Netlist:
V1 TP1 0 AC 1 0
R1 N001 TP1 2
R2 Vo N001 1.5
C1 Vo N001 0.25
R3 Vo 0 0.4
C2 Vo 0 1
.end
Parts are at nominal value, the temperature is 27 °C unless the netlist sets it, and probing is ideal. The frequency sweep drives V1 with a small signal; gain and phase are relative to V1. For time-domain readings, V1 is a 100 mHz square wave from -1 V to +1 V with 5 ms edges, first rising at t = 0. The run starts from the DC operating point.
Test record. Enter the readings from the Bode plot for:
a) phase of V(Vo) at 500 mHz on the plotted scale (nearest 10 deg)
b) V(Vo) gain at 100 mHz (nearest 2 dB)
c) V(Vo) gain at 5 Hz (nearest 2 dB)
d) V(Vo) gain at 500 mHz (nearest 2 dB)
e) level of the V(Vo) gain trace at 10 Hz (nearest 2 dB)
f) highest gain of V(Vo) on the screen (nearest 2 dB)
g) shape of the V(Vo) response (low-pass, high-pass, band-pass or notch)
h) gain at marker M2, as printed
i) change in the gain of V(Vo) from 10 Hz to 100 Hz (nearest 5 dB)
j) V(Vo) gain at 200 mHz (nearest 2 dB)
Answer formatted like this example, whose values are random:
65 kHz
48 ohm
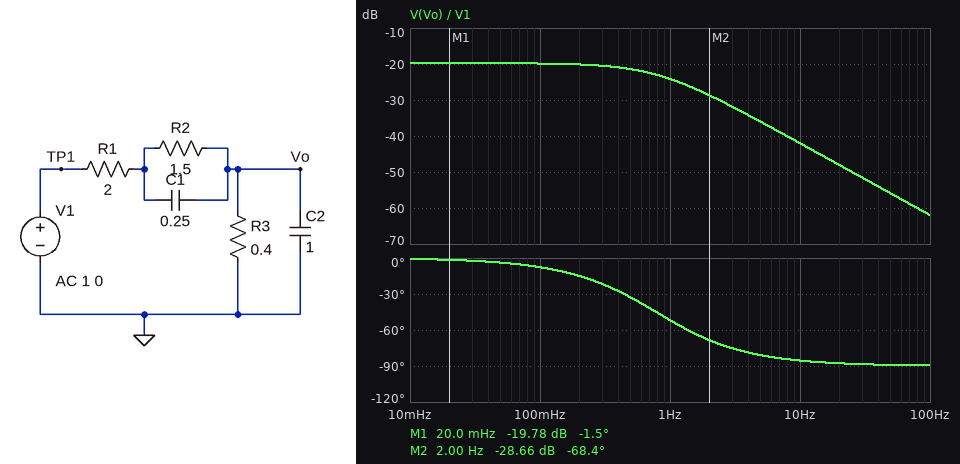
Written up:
-30 deg
-20 dB
-36 dB
-22 dB
-42 dB
-20 dB
low-pass
-28.66 dB
-20 dB
-20 dB
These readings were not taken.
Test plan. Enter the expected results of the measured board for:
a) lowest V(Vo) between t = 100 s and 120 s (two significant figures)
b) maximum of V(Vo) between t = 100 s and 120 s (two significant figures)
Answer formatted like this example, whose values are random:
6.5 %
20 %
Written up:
-100 mV
100 mV
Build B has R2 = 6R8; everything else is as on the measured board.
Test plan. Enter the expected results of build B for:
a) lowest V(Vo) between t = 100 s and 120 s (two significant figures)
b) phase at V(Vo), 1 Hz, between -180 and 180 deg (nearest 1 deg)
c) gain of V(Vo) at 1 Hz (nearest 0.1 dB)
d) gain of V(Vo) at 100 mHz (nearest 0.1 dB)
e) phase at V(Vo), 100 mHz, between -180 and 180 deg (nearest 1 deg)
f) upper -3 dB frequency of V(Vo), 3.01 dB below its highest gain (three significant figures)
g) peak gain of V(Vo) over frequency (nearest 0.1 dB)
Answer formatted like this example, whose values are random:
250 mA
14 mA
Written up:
-120 mV
-48 deg
-23.6 dB
-24.6 dB
18 deg
1.02 Hz
-20.7 dB
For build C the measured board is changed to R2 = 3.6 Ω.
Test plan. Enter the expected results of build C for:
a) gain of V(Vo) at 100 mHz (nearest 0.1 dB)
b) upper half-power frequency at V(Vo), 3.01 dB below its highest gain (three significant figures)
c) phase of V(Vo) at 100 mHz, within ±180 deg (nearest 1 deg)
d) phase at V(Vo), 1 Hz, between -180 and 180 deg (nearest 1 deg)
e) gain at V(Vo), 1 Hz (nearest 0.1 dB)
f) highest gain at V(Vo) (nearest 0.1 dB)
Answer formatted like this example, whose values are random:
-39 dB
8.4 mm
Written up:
-22.8 dB
1.04 Hz
4 deg
-49 deg
-23.8 dB
-21.0 dB
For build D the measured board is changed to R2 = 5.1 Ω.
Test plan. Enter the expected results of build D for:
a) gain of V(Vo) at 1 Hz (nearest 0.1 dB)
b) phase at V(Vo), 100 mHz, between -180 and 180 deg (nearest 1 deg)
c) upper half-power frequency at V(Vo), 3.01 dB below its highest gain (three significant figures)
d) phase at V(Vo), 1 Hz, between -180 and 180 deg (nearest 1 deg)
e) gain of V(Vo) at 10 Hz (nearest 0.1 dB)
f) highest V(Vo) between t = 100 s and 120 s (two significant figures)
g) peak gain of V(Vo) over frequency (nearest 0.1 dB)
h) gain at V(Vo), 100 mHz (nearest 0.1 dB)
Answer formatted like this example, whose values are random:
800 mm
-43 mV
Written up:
-23.7 dB
11 deg
1.03 Hz
-49 deg
-42.0 dB
110 mV
-20.9 dB
-23.9 dB
